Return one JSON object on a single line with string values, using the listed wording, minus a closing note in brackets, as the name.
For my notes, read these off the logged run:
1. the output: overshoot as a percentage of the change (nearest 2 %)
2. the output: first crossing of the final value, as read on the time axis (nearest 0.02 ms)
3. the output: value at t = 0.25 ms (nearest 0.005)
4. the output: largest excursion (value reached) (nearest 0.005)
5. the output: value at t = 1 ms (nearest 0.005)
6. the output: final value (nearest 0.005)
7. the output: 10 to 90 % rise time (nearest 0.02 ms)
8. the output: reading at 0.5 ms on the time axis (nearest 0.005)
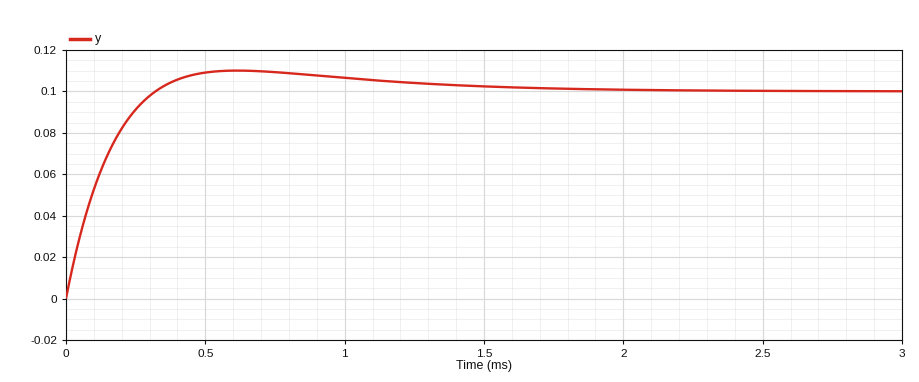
{"the output: overshoot as a percentage of the change": "10 %", "the output: first crossing of the final value, as read on the time axis": "0.32 ms", "the output: value at t = 0.25 ms": "0.090", "the output: largest excursion (value reached)": "0.110", "the output: value at t = 1 ms": "0.105", "the output: final value": "0.100", "the output: 10 to 90 % rise time": "0.22 ms", "the output: reading at 0.5 ms on the time axis": "0.110"}
